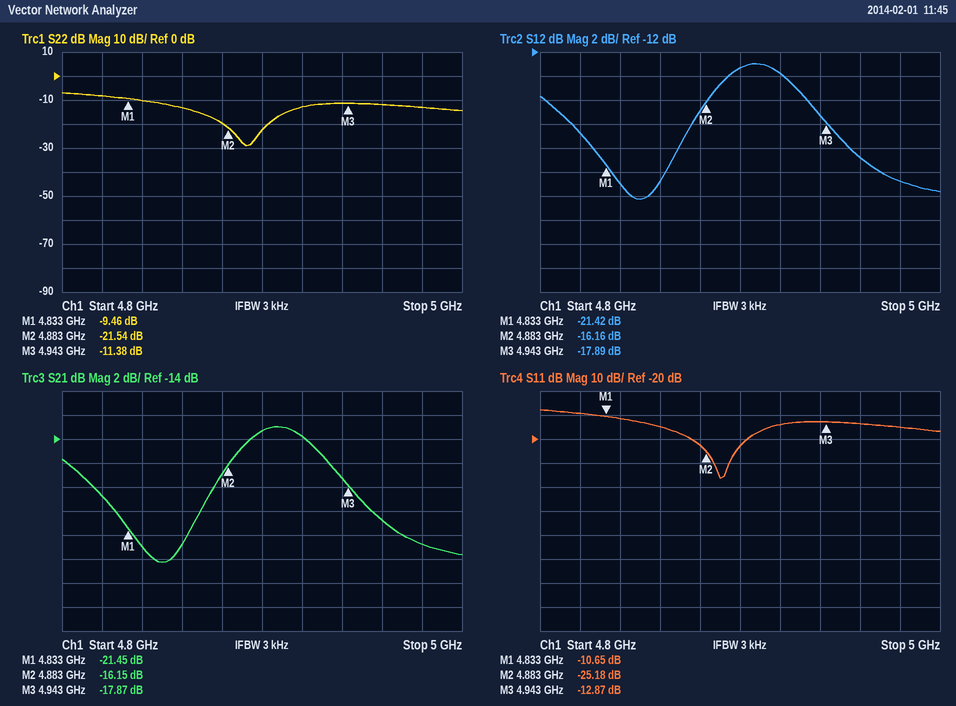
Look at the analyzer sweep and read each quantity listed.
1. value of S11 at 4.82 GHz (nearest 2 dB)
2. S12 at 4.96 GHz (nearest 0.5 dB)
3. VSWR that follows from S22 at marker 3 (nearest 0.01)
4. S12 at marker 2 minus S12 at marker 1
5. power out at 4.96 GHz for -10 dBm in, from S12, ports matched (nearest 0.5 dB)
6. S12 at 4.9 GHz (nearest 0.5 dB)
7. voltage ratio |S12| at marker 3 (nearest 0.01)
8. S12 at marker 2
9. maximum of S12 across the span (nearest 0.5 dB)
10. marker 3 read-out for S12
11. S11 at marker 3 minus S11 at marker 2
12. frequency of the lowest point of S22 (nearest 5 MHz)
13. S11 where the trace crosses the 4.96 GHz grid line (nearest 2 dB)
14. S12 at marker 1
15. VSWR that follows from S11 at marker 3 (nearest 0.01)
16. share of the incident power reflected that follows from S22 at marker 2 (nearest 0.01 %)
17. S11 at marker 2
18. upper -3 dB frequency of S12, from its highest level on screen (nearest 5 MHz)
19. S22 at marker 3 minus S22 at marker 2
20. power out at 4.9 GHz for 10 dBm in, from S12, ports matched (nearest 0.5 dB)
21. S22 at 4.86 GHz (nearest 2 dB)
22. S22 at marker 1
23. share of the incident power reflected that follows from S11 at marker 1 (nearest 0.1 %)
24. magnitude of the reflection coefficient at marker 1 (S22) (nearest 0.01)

-10 dB
-21.0 dB
1.74
5.26 dB
-31.0 dBm
-13.5 dB
0.13
-16.16 dB
-13.0 dB
-17.89 dB
12.31 dB
4.890 GHz
-14 dB
-21.42 dB
1.59
0.70 %
-25.18 dB
4.935 GHz
10.16 dB
-3.5 dBm
-14 dB
-9.46 dB
8.6 %
0.34
